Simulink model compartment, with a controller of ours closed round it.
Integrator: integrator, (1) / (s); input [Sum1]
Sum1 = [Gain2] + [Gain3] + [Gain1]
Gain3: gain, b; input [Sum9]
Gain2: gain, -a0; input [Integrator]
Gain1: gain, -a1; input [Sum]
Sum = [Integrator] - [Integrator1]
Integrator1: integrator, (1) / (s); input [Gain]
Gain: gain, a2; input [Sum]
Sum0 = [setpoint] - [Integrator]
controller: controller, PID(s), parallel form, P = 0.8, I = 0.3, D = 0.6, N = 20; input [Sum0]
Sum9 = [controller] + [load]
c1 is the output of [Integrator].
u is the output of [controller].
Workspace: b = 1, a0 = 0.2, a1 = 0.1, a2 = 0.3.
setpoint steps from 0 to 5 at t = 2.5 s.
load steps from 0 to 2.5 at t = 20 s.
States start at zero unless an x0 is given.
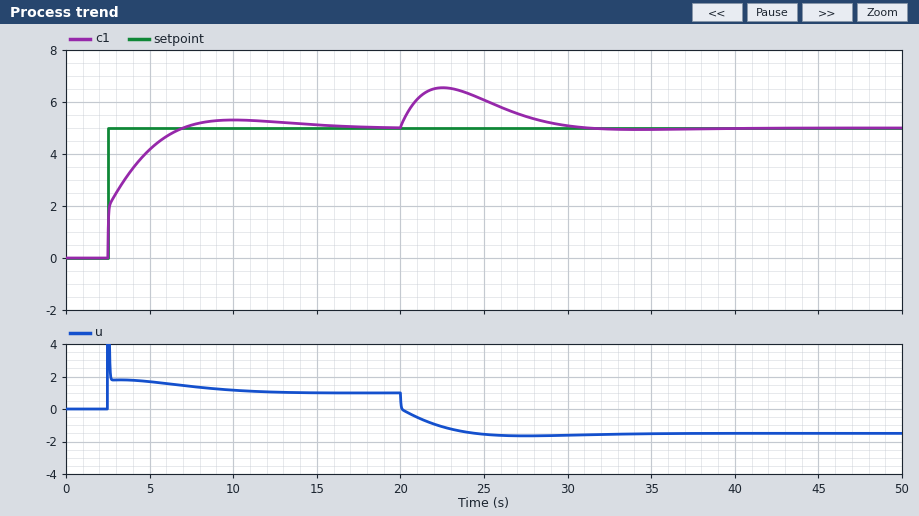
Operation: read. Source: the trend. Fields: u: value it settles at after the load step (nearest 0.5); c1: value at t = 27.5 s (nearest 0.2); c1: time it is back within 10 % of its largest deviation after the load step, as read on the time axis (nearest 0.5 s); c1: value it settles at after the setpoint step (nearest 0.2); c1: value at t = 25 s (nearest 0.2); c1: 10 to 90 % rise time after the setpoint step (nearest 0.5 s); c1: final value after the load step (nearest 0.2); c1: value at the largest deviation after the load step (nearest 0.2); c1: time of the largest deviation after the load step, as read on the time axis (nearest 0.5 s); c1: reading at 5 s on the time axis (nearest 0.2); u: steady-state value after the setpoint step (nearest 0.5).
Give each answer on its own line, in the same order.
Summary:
-1.5
5.4
29.5 s
5.0
6.0
3.0 s
5.0
6.6
22.5 s
4.2
1.0
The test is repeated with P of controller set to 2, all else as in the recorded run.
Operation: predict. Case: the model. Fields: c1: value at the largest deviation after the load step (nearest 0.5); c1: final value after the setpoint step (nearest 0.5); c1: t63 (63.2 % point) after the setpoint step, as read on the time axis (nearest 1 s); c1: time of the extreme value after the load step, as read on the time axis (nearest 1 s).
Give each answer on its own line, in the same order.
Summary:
6.0
5.0
3 s
22 s
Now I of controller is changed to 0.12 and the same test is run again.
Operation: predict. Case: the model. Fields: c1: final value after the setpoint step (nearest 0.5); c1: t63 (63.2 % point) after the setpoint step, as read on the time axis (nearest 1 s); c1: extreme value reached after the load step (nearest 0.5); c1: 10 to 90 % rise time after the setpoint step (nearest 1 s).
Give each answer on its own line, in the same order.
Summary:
5.0
4 s
7.0
5 s
